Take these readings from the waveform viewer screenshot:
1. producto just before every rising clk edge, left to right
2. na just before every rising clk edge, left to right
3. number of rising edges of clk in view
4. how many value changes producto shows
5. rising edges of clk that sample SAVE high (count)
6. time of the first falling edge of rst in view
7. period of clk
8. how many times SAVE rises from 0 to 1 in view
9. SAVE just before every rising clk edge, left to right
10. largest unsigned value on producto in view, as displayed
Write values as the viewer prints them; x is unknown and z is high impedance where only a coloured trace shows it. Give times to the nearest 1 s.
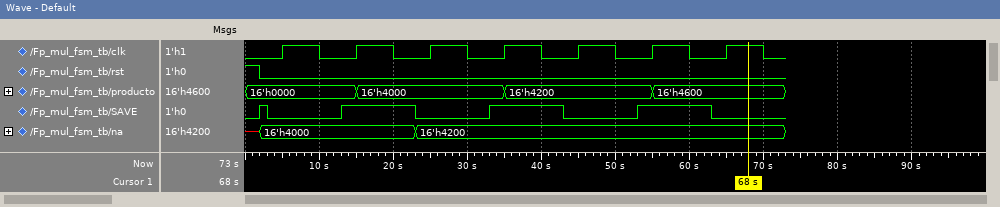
16'h0000, 16'h0000, 16'h4000, 16'h4000, 16'h4200, 16'h4200, 16'h4600
16'h4000, 16'h4000, 16'h4200, 16'h4200, 16'h4200, 16'h4200, 16'h4200
7
3
3
2 s
10 s
4
0 1 0 1 0 1 0
16'h4600
